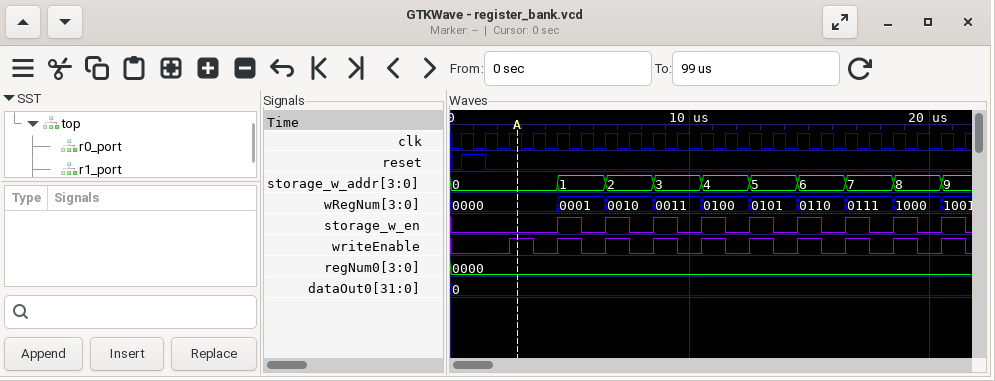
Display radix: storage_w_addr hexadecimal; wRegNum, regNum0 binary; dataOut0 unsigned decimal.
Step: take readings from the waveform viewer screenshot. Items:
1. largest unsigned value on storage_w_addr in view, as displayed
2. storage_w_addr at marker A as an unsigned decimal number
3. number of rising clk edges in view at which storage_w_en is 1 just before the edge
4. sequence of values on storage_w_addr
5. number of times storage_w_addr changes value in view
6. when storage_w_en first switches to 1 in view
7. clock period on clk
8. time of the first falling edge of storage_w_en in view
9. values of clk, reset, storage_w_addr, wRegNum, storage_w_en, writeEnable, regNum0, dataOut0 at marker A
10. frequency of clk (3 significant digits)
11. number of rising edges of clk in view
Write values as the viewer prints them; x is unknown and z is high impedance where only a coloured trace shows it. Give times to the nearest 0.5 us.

9
0
9
0, 1, 2, 3, 4, 5, 6, 7, 8, 9
9
4.5 us
1 us
5.5 us
clk=1, reset=0, storage_w_addr=0, wRegNum=0000, storage_w_en=0, writeEnable=1, regNum0=0000, dataOut0=0
1.00 MHz
22
